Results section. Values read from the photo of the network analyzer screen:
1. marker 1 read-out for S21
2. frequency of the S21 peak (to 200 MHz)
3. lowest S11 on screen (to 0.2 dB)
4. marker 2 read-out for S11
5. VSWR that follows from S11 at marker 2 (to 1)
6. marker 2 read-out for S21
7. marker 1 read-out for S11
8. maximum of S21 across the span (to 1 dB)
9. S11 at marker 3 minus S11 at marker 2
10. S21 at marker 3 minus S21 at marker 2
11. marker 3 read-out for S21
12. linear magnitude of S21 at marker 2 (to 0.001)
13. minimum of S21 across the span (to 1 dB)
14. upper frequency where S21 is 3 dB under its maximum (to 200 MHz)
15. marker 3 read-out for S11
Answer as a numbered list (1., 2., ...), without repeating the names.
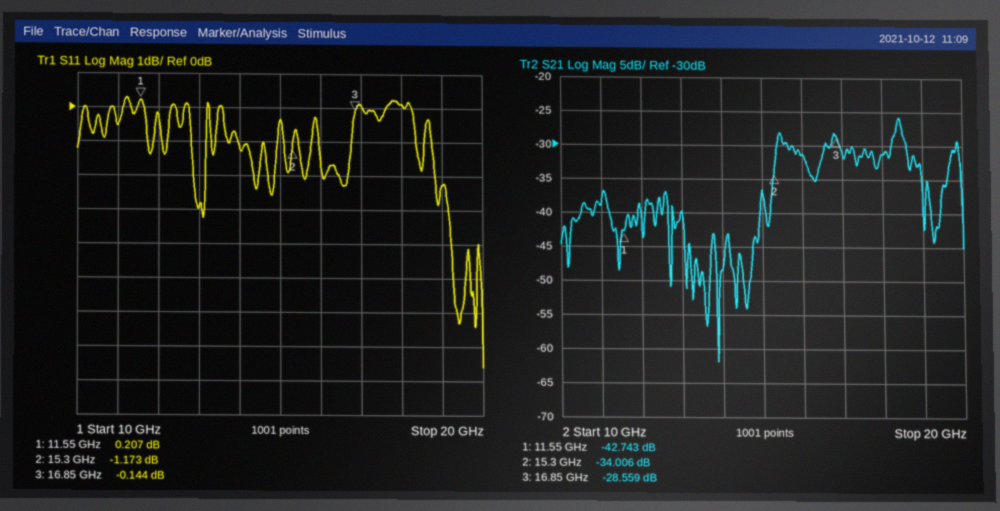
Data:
1. -42.743 dB
2. 18.4 GHz
3. -7.6 dB
4. -1.173 dB
5. 15
6. -34.006 dB
7. 0.207 dB
8. -26 dB
9. 1.029 dB
10. 5.447 dB
11. -28.559 dB
12. 0.020
13. -62 dB
14. 18.6 GHz
15. -0.144 dB
